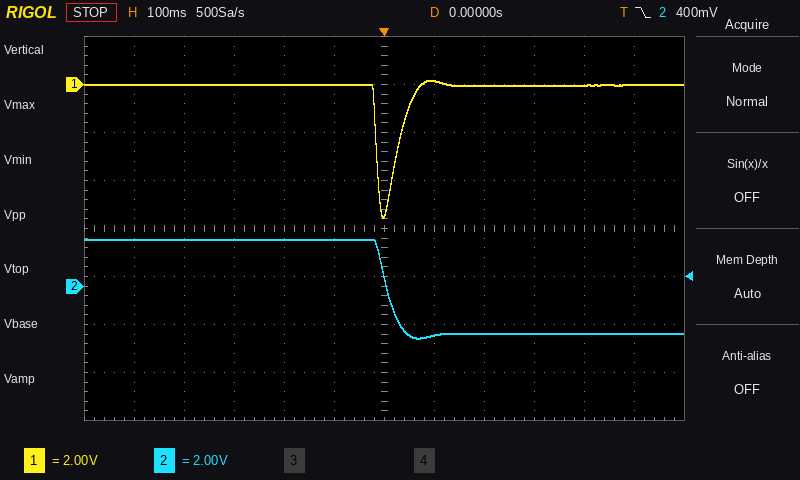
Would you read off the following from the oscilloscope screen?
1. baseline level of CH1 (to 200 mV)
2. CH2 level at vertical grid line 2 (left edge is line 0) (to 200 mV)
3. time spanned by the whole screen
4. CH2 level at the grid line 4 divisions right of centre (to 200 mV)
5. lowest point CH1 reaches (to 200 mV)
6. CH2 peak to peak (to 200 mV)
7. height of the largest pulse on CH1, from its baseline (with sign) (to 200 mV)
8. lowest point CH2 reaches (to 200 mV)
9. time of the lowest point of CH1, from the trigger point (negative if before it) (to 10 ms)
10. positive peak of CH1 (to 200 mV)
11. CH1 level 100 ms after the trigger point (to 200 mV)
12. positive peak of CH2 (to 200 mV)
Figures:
0.0 V
2.0 V
1.2 s
-2.0 V
-5.6 V
4.2 V
-5.6 V
-2.2 V
0 ms
200 mV
200 mV
2.0 V
